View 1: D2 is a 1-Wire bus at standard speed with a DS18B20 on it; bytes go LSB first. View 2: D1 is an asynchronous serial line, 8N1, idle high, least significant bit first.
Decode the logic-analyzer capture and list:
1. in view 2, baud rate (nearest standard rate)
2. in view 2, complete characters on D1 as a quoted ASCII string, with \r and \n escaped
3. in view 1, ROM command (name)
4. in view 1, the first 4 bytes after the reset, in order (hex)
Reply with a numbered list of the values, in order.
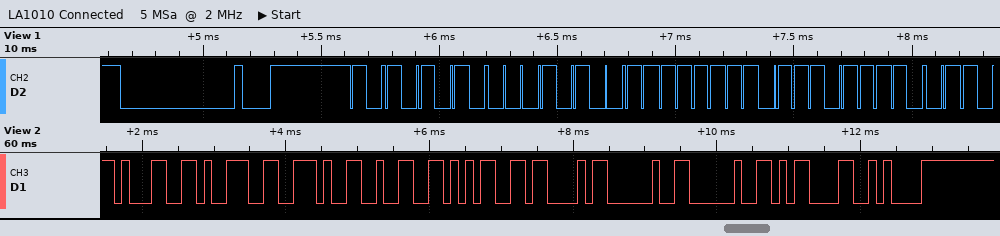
1. 9600 baud
2. "19.25C  \r\n"
3. Match ROM
4. 55 28 FF EE
